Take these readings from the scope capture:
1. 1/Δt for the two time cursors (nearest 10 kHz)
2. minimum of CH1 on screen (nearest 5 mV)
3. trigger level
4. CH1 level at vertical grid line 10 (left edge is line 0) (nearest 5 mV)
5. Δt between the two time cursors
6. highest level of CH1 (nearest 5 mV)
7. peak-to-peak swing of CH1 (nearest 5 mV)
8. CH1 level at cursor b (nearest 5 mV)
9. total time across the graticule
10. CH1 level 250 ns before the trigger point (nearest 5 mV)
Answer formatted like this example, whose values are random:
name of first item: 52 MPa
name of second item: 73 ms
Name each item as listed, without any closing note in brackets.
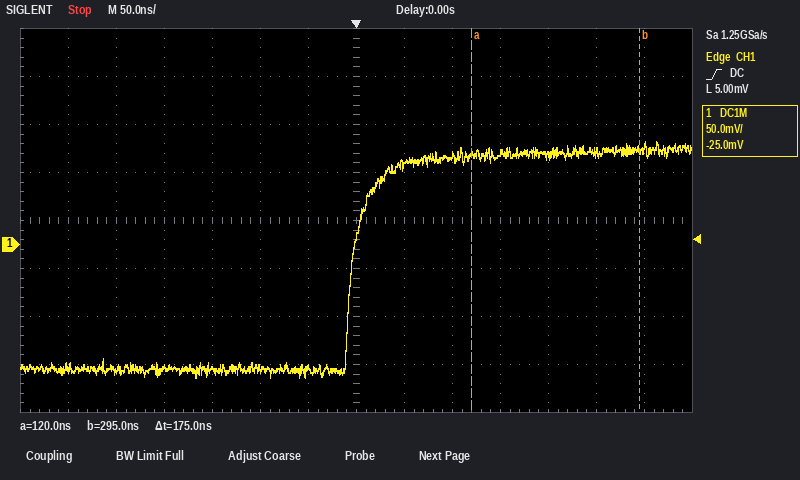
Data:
1/Δt for the two time cursors: 5.71 MHz
minimum of CH1 on screen: -140 mV
trigger level: 5.00 mV
CH1 level at vertical grid line 10 (left edge is line 0): 95 mV
Δt between the two time cursors: 175 ns
highest level of CH1: 105 mV
peak-to-peak swing of CH1: 245 mV
CH1 level at cursor b: 100 mV
total time across the graticule: 700 ns
CH1 level 250 ns before the trigger point: -130 mV
